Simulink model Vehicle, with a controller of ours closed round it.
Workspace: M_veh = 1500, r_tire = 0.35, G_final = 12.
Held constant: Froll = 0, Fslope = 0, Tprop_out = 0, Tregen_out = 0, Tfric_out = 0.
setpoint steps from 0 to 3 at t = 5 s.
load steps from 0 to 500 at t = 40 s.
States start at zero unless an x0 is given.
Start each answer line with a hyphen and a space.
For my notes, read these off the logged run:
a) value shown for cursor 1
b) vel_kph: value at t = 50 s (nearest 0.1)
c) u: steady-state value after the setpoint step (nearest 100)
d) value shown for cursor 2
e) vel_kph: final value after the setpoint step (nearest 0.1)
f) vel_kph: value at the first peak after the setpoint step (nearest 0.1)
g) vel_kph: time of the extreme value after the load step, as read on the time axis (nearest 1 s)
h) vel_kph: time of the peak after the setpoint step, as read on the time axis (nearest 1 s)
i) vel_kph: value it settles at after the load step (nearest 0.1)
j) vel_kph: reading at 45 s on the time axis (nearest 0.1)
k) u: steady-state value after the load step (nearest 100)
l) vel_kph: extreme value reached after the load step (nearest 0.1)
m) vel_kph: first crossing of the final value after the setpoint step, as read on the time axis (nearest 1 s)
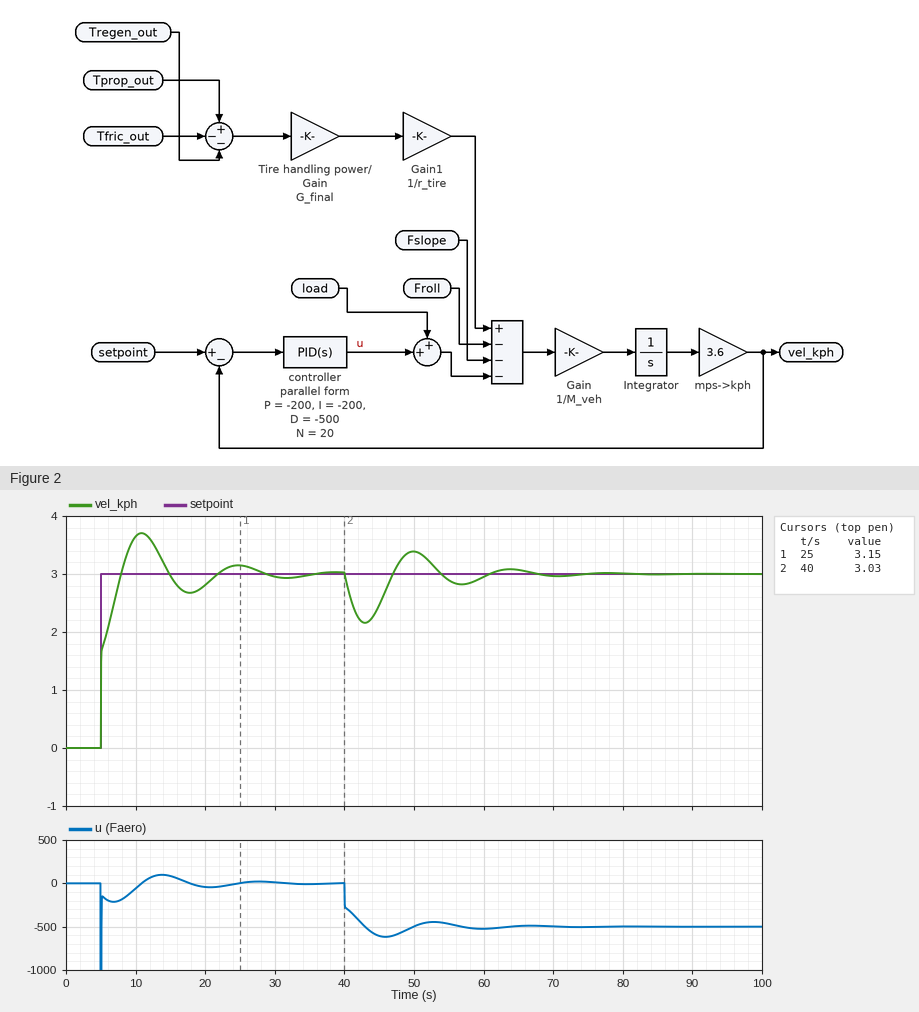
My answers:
- 3.15
- 3.4
- 0
- 3.03
- 3.0
- 3.7
- 43 s
- 11 s
- 3.0
- 2.5
- -500
- 2.2
- 8 s
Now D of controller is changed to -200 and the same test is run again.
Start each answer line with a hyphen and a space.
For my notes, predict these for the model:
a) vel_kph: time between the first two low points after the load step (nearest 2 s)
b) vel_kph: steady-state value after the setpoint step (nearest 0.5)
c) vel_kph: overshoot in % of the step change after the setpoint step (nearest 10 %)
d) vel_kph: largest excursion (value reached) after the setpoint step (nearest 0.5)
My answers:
- 12 s
- 3.0
- 30 %
- 4.0
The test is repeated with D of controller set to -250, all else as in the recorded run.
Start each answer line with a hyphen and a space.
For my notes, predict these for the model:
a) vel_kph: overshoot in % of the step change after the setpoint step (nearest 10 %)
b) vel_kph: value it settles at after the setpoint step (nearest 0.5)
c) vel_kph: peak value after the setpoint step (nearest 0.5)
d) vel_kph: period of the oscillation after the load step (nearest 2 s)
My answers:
- 30 %
- 3.0
- 4.0
- 12 s
